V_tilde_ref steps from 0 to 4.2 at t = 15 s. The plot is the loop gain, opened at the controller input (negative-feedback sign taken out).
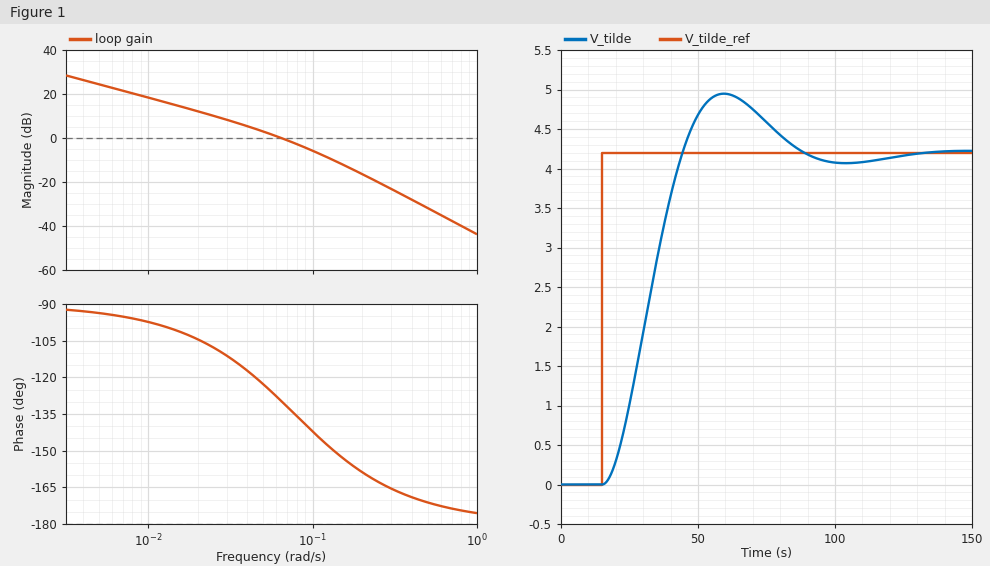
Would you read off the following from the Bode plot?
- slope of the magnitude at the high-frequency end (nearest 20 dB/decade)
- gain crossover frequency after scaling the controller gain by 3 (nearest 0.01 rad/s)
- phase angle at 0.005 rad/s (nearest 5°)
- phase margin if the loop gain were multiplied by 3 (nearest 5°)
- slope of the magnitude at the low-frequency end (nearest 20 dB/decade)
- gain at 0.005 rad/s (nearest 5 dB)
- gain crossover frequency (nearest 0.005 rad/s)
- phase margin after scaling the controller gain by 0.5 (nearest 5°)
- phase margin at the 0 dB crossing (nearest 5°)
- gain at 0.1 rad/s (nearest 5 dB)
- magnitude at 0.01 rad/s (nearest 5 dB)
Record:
-40 dB/decade
0.13 rad/s
-95°
30°
-20 dB/decade
25 dB
0.065 rad/s
65°
50°
-5 dB
20 dB
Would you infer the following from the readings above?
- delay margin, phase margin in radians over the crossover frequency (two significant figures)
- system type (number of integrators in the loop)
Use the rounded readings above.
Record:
13 s
1
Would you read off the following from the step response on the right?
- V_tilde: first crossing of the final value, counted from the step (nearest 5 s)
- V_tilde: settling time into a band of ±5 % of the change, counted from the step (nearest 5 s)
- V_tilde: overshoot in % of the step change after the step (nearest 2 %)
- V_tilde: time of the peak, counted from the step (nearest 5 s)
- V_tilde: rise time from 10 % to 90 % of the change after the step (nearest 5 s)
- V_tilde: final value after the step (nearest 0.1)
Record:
30 s
65 s
18 %
45 s
20 s
4.2
